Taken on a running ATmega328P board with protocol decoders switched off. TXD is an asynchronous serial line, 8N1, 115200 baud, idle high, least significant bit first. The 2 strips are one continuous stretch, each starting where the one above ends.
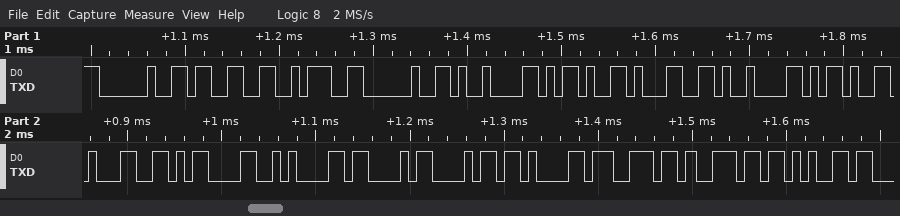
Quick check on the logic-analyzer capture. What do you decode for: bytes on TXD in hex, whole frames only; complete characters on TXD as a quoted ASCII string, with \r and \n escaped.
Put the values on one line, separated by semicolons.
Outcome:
20 33 3A 20 09 2D 31 09 2D 31 0D 0A 43 68 61 6E 6E 65; " 3: \t-1\t-1\r\nChanne"
